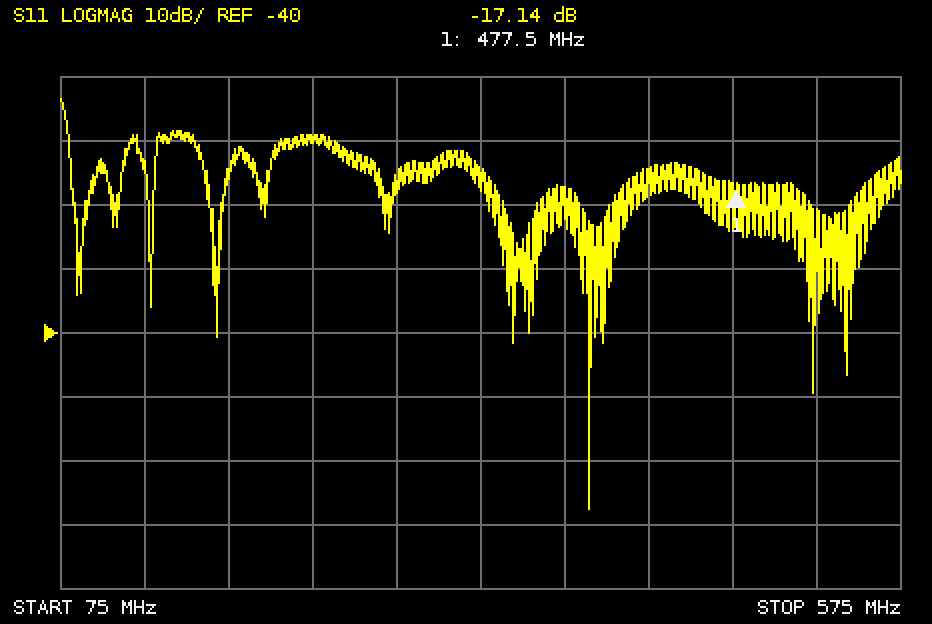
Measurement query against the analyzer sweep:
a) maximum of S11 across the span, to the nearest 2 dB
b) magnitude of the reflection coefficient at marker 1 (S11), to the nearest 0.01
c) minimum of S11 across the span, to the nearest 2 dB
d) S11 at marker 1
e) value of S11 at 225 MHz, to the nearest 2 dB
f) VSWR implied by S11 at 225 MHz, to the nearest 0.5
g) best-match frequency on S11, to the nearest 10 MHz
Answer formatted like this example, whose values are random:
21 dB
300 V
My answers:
-4 dB
0.14
-68 dB
-17.14 dB
-10 dB
2.0
390 MHz
